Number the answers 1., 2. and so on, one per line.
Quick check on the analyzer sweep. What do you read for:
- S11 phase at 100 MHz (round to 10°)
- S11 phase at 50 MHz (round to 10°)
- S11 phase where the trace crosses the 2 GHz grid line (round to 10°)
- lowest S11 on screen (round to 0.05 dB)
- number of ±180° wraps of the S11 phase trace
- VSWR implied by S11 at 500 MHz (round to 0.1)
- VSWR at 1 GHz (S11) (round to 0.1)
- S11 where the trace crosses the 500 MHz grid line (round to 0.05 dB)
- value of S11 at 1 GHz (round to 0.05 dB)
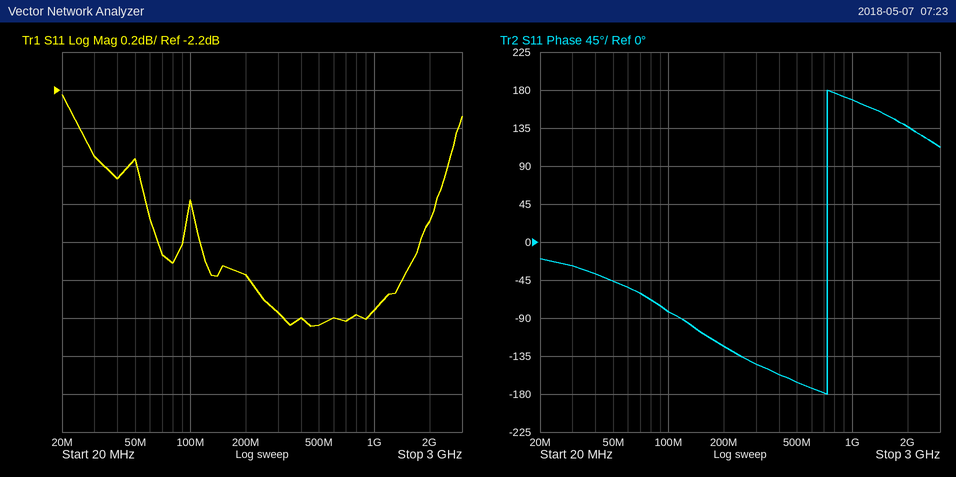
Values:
1. -80°
2. -50°
3. 140°
4. -3.45 dB
5. 1
6. 5.1
7. 5.2
8. -3.45 dB
9. -3.35 dB
